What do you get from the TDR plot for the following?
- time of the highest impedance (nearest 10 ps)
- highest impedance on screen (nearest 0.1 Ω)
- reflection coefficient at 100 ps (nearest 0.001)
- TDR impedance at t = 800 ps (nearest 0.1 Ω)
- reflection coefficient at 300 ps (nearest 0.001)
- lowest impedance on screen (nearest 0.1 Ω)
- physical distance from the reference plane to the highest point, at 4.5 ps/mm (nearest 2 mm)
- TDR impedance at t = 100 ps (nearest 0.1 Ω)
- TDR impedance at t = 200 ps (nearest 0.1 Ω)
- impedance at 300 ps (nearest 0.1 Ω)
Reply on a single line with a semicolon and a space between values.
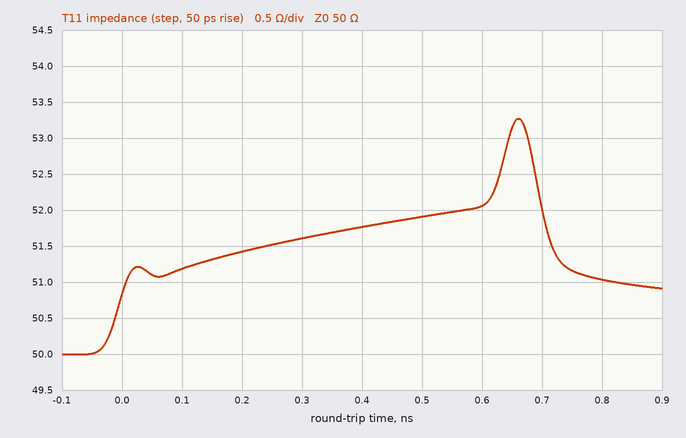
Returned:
660 ps; 53.3 Ω; +0.012; 51.0 Ω; +0.016; 50.0 Ω; 74 mm; 51.2 Ω; 51.4 Ω; 51.6 Ω
